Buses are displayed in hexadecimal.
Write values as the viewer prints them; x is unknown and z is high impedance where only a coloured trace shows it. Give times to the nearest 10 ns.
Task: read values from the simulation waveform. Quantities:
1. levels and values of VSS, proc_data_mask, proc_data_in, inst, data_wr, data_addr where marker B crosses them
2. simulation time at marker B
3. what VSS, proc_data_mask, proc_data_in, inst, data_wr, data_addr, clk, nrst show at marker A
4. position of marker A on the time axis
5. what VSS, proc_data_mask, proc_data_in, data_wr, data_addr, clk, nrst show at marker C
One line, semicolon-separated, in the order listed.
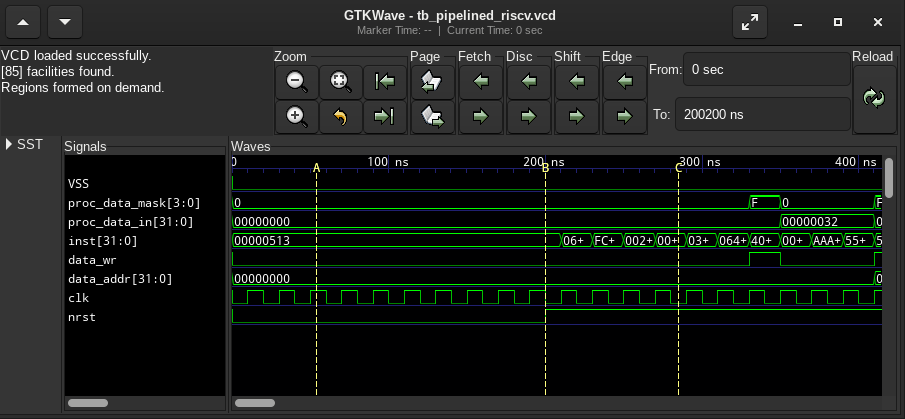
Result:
VSS=0, proc_data_mask=0, proc_data_in=00000000, inst=00000513, data_wr=0, data_addr=00000000; 200 ns; VSS=0, proc_data_mask=0, proc_data_in=00000000, inst=00000513, data_wr=0, data_addr=00000000, clk=1, nrst=0; 50 ns; VSS=0, proc_data_mask=0, proc_data_in=00000000, data_wr=0, data_addr=00000000, clk=0, nrst=1
